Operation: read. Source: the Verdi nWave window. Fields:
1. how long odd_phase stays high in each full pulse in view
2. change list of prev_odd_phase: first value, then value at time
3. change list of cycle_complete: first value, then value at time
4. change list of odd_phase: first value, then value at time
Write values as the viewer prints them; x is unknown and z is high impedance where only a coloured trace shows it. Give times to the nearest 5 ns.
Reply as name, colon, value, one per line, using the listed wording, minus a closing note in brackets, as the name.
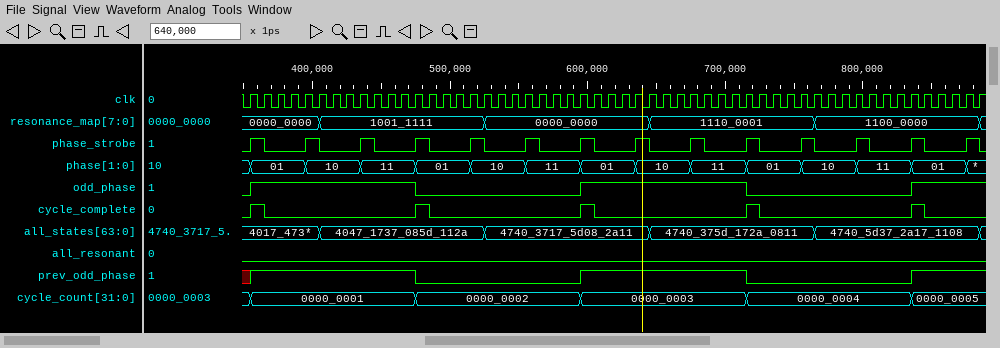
how long odd_phase stays high in each full pulse in view: 120 ns, 120 ns
change list of prev_odd_phase: first value, then value at time: x, 1 at 355 ns, 0 at 475 ns, 1 at 595 ns, 0 at 715 ns, 1 at 835 ns
change list of cycle_complete: first value, then value at time: 0, 1 at 355 ns, 0 at 365 ns, 1 at 475 ns, 0 at 485 ns, 1 at 595 ns, 0 at 605 ns, 1 at 715 ns, 0 at 725 ns, 1 at 835 ns, 0 at 845 ns
change list of odd_phase: first value, then value at time: 0, 1 at 355 ns, 0 at 475 ns, 1 at 595 ns, 0 at 715 ns, 1 at 835 ns
